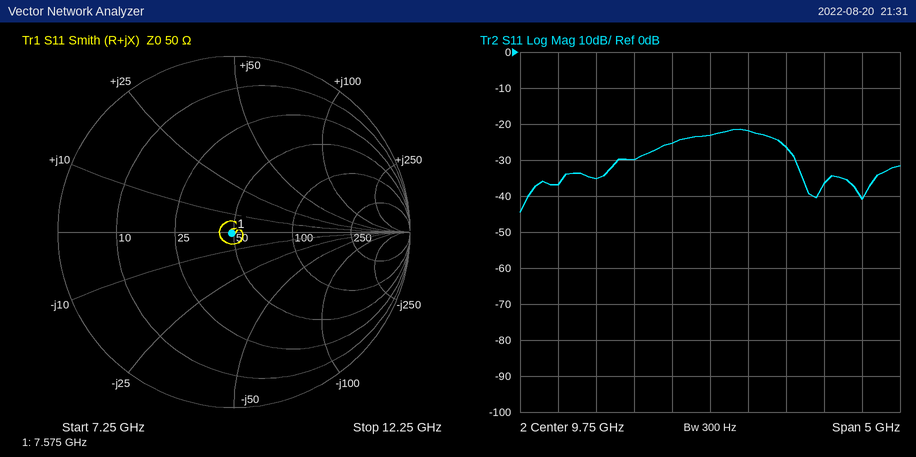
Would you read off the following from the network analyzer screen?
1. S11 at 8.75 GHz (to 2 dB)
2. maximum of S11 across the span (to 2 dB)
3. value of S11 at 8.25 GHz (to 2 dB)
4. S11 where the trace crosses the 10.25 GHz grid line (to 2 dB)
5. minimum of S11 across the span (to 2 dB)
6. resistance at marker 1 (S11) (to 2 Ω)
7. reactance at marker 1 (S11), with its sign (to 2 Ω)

-30 dB
-22 dB
-36 dB
-22 dB
-44 dB
48 Ω
0 Ω
